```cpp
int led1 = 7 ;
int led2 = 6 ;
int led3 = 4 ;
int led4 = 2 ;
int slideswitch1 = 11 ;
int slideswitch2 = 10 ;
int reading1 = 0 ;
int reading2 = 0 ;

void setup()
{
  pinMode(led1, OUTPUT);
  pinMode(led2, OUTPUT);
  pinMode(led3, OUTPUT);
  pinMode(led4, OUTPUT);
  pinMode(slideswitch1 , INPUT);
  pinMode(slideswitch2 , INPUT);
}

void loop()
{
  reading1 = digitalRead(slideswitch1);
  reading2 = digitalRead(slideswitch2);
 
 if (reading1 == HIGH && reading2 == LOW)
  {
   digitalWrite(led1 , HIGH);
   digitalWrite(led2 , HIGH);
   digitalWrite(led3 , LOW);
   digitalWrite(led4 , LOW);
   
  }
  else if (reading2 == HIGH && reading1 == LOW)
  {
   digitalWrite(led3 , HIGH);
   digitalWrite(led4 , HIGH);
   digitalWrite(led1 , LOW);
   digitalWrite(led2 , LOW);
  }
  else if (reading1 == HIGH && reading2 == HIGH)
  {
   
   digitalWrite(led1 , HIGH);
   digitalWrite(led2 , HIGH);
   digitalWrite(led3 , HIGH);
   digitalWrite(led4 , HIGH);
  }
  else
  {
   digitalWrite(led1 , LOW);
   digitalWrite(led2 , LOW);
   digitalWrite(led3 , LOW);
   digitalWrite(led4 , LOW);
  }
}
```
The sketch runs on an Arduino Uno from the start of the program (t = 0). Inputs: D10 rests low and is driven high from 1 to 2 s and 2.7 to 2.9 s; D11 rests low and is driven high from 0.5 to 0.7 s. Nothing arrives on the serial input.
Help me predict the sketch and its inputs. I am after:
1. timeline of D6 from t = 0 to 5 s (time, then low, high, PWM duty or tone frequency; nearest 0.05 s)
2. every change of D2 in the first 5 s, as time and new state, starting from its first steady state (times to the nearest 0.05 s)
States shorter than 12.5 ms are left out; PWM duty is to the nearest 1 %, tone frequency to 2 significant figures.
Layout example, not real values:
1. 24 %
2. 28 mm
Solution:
1. 0 s low; 0.5 s high; 0.7 s low
2. 0 s low; 1 s high; 2 s low; 2.7 s high; 2.9 s low
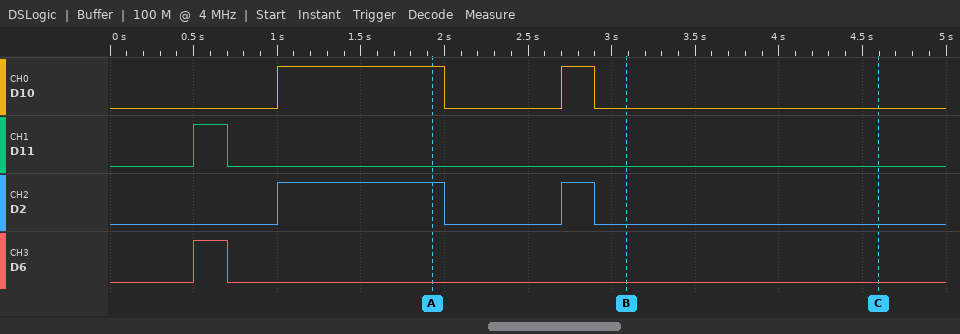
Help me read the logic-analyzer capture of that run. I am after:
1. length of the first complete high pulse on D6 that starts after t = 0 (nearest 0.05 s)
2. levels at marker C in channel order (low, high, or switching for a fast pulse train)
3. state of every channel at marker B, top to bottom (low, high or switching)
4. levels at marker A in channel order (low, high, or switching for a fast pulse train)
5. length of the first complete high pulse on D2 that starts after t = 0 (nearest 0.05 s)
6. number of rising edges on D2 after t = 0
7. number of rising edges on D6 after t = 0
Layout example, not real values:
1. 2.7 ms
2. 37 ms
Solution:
1. 0.20 s
2. D10 low, D11 low, D2 low, D6 low
3. D10 low, D11 low, D2 low, D6 low
4. D10 high, D11 low, D2 high, D6 low
5. 1.00 s
6. 2
7. 1
